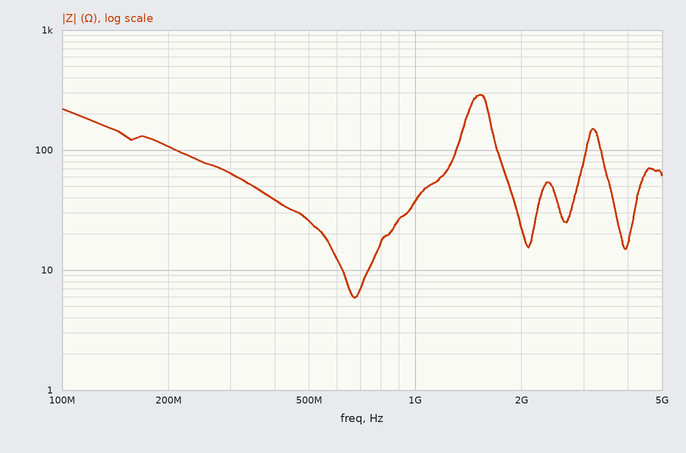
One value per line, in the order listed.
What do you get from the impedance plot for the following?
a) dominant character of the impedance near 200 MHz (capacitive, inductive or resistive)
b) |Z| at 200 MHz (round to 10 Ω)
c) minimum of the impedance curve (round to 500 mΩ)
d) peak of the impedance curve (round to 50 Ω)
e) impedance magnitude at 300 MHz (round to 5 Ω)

capacitive
110 Ω
6.0 Ω
300 Ω
65 Ω
